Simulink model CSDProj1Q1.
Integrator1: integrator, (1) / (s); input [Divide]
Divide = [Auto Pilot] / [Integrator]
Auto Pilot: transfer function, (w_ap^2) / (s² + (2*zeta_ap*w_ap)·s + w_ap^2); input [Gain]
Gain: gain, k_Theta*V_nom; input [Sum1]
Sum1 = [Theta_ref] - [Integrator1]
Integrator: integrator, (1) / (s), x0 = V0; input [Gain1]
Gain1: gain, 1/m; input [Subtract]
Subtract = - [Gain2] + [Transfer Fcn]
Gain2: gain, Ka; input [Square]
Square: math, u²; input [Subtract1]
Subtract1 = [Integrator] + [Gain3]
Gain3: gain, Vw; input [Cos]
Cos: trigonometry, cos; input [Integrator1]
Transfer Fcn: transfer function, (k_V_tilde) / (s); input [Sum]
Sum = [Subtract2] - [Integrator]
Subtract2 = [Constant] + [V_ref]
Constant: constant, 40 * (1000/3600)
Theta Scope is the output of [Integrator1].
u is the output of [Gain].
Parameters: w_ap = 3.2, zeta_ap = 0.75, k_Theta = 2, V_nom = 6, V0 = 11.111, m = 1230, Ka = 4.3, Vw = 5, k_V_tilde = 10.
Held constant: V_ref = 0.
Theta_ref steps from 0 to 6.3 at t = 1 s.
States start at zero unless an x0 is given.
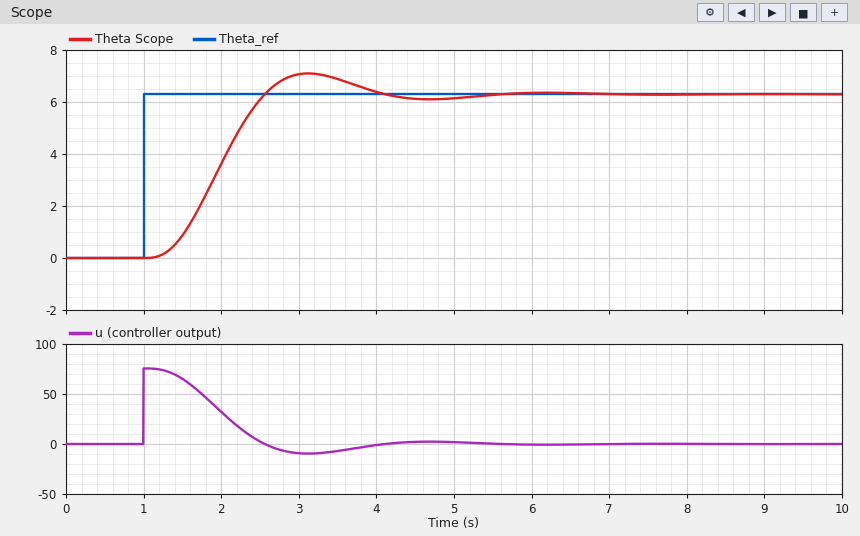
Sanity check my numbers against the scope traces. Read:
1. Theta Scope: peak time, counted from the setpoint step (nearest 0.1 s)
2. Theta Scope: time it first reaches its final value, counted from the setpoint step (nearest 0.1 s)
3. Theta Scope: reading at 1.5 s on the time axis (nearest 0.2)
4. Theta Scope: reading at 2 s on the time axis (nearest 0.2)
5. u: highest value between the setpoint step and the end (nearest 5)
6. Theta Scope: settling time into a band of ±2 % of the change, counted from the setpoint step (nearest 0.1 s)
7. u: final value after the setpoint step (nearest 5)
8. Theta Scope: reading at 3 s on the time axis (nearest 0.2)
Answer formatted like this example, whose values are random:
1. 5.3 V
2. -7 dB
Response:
1. 2.1 s
2. 1.6 s
3. 0.8
4. 3.6
5. 75
6. 4.1 s
7. 0
8. 7.0
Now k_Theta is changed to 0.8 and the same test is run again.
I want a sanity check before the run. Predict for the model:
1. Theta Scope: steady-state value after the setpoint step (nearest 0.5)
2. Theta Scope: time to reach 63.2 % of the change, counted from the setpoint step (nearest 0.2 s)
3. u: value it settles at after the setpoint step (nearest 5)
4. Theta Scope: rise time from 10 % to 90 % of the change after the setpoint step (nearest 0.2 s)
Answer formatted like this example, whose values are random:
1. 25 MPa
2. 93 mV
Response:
1. 6.5
2. 2.0 s
3. 0
4. 3.2 s
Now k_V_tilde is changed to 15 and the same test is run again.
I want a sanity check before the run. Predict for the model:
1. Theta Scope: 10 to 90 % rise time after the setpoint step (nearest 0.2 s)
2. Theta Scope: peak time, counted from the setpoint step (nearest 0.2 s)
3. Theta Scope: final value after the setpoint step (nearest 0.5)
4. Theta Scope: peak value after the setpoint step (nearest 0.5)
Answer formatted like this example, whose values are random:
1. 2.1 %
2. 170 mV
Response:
1. 1.0 s
2. 2.2 s
3. 6.5
4. 7.0
